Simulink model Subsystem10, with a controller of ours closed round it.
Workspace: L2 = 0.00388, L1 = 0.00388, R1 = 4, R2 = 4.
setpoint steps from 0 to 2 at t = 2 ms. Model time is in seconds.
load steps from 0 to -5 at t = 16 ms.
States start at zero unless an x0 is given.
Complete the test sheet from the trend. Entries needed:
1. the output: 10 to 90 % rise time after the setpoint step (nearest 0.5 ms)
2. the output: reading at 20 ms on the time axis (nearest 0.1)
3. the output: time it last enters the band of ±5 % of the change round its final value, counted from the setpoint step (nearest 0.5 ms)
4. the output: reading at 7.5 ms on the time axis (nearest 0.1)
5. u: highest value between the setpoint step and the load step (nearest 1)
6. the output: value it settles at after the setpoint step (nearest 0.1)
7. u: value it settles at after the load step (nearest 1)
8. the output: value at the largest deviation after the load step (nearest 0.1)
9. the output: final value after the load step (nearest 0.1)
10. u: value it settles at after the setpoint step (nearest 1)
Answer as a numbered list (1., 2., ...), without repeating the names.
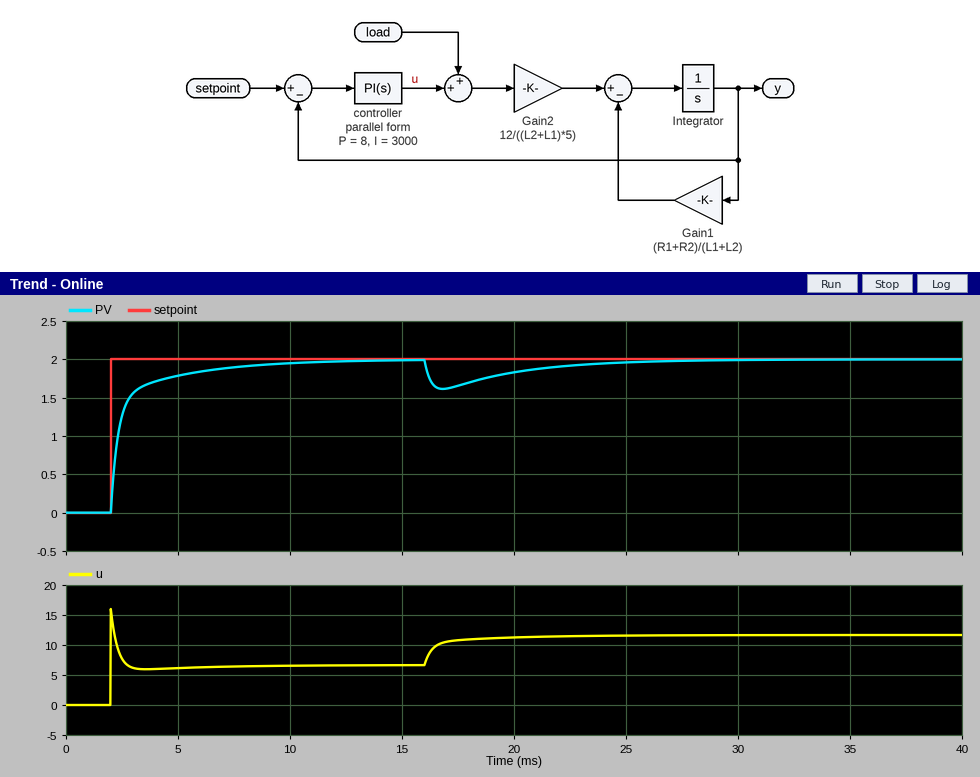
1. 3.0 ms
2. 1.8
3. 5.5 ms
4. 1.9
5. 16
6. 2.0
7. 12
8. 1.6
9. 2.0
10. 7
